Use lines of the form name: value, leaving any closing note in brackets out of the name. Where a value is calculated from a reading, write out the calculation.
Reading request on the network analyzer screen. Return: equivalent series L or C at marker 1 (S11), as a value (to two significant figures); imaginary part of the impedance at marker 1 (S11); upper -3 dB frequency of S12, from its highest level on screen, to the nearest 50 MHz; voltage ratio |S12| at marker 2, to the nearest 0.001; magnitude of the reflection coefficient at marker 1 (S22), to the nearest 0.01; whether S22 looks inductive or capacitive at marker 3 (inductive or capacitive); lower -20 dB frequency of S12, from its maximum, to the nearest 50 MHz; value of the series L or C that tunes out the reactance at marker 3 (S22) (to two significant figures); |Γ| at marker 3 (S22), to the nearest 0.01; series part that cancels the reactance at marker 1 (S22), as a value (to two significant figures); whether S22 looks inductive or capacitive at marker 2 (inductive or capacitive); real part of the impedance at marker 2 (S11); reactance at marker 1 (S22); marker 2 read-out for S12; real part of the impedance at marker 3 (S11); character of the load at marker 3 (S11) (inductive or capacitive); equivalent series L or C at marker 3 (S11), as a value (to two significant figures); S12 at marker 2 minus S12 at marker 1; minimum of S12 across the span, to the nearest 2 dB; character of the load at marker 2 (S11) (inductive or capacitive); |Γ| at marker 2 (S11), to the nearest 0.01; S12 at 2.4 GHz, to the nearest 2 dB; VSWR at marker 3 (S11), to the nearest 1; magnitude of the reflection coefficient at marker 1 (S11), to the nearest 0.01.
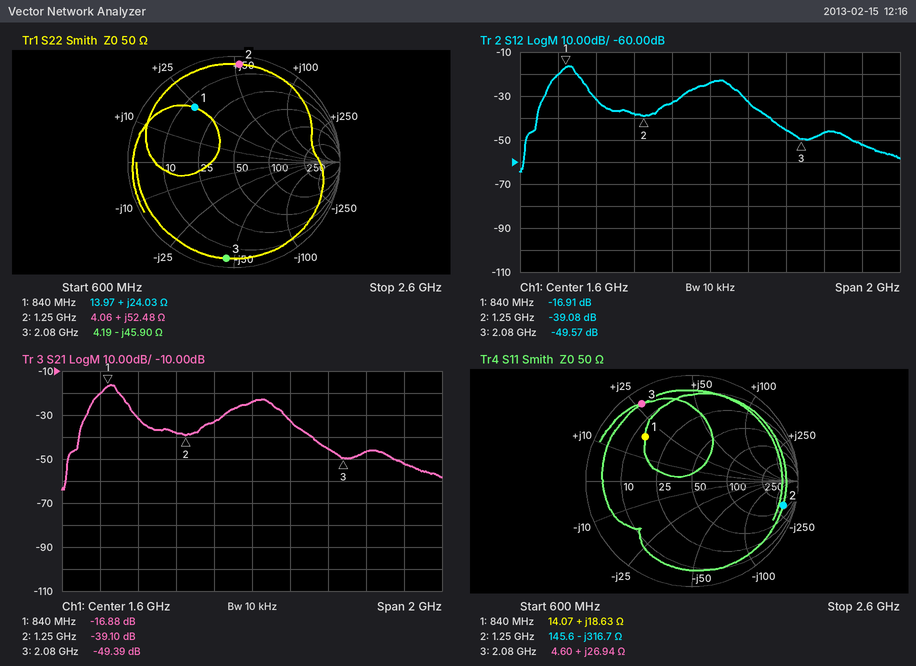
equivalent series L or C at marker 1 (S11), as a value: L = 18.63 Ω/(2π × 840 MHz) ≈ 3.5 nH
imaginary part of the impedance at marker 1: +18.63 Ω
upper -3 dB frequency of S12, from its highest level on screen, to the nearest 50 MHz: 900 MHz
voltage ratio |S12| at marker 2, to the nearest 0.001: 10^(-39.08/20) ≈ 0.011
magnitude of the reflection coefficient at marker 1 (S22), to the nearest 0.01: 0.63
whether S22 looks inductive or capacitive at marker 3: capacitive
lower -20 dB frequency of S12, from its maximum, to the nearest 50 MHz: 700 MHz
value of the series L or C that tunes out the reactance at marker 3 (S22): L = 45.9 Ω/(2π × 2.08 GHz) ≈ 3.5 nH
|Γ| at marker 3 (S22), to the nearest 0.01: 0.91
series part that cancels the reactance at marker 1 (S22), as a value: C = 1/(2π × 840 MHz × 24.03 Ω) ≈ 7.9 pF
whether S22 looks inductive or capacitive at marker 2: inductive
real part of the impedance at marker 2: 145.6 Ω
reactance at marker 1: +24.03 Ω
marker 2 read-out for S12: -39.08 dB
real part of the impedance at marker 3: 4.60 Ω
character of the load at marker 3 (S11): inductive
equivalent series L or C at marker 3 (S11), as a value: L = 26.94 Ω/(2π × 2.08 GHz) ≈ 2.1 nH
S12 at marker 2 minus S12 at marker 1: -39.08 − (-16.91) = -22.17 dB
minimum of S12 across the span, to the nearest 2 dB: -64 dB
character of the load at marker 2 (S11): capacitive
|Γ| at marker 2 (S11), to the nearest 0.01: 0.89
S12 at 2.4 GHz, to the nearest 2 dB: -52 dB
VSWR at marker 3 (S11), to the nearest 1: 14
magnitude of the reflection coefficient at marker 1 (S11), to the nearest 0.01: 0.61
